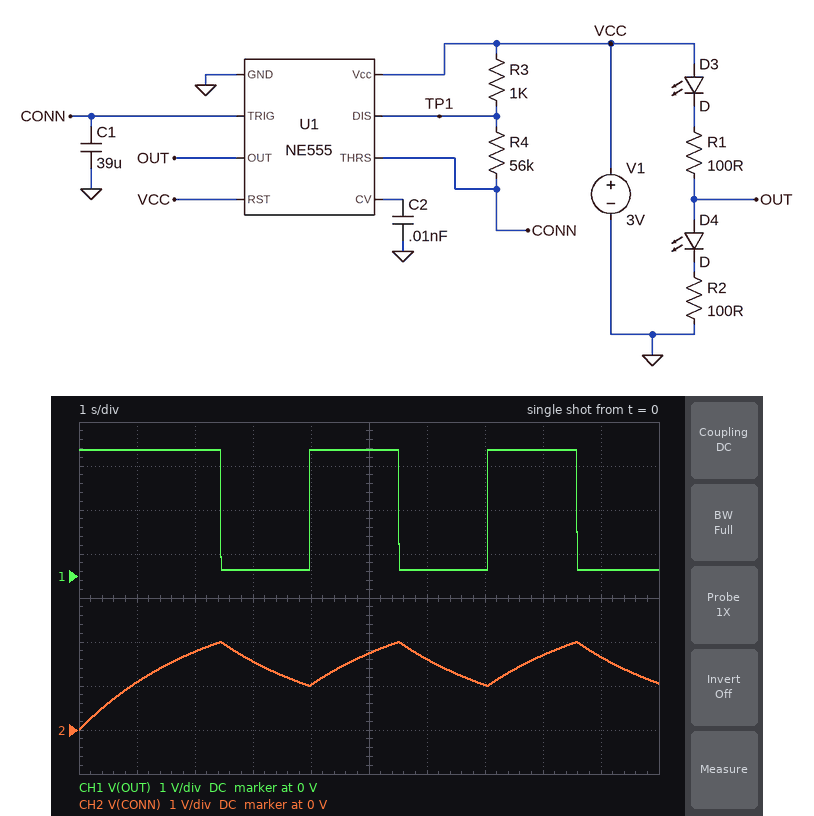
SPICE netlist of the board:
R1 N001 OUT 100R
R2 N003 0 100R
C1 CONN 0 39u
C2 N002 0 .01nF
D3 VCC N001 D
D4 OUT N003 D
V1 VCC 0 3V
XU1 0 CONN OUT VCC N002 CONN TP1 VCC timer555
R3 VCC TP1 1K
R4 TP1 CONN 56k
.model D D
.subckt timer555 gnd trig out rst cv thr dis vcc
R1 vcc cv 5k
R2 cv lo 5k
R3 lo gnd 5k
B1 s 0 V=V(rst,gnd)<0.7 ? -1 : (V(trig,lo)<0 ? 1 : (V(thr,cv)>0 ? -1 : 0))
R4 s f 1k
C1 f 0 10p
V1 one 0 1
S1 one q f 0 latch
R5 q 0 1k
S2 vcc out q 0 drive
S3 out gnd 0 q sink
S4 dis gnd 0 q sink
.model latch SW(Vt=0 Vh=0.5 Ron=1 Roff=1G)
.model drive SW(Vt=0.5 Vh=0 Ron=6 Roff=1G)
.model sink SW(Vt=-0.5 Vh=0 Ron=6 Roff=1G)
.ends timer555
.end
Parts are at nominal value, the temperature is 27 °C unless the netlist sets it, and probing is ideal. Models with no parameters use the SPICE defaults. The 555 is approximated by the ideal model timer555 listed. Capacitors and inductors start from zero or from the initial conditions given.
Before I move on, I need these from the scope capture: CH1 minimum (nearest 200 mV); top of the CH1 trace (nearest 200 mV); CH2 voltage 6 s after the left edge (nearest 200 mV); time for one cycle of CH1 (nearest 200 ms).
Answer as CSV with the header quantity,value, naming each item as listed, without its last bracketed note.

quantity,value
CH1 minimum,200 mV
top of the CH1 trace,2.8 V
CH2 voltage 6 s after the left edge,1.6 V
time for one cycle of CH1,3.0 s
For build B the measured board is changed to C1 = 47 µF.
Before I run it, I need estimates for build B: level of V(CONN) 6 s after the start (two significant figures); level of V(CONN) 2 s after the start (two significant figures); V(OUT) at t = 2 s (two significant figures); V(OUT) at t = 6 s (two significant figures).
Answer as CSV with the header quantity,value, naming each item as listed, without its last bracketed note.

quantity,value
level of V(CONN) 6 s after the start,1.7 V
level of V(CONN) 2 s after the start,1.6 V
V(OUT) at t = 2 s,2.9 V
V(OUT) at t = 6 s,2.9 V
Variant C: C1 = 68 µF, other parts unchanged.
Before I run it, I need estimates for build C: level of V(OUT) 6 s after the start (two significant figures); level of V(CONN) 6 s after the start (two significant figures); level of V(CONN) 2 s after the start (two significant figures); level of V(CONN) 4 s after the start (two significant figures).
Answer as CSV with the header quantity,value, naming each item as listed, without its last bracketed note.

quantity,value
level of V(OUT) 6 s after the start,130 mV
level of V(CONN) 6 s after the start,1.3 V
level of V(CONN) 2 s after the start,1.2 V
level of V(CONN) 4 s after the start,1.9 V
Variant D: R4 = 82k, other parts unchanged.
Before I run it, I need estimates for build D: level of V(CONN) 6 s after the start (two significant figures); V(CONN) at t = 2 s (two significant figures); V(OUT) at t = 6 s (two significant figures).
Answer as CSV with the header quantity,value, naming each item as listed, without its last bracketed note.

quantity,value
level of V(CONN) 6 s after the start,1.1 V
V(CONN) at t = 2 s,1.4 V
V(OUT) at t = 6 s,2.9 V
